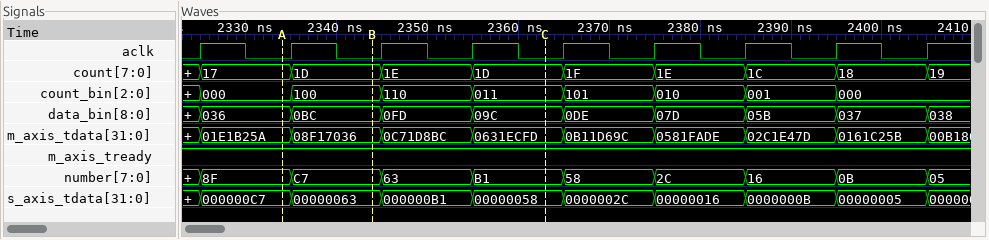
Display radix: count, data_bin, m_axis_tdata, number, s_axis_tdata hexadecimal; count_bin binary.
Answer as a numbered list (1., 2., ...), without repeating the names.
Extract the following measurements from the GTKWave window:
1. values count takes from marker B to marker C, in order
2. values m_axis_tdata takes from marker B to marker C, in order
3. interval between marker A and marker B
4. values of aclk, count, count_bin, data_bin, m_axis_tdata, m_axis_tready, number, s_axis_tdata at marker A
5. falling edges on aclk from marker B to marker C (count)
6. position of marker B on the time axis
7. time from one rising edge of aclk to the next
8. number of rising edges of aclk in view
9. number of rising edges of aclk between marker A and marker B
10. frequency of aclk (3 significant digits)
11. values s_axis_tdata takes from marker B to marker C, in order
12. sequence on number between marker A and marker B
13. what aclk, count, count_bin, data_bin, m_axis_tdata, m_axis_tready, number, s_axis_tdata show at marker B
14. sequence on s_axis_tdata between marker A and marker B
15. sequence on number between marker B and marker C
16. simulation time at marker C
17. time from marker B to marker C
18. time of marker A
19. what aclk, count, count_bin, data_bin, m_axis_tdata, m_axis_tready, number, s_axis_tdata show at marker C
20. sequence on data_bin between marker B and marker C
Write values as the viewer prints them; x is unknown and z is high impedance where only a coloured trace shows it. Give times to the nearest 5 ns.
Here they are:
1. 1D, 1E, 1D
2. 08F17036, 0C71D8BC, 0631ECFD
3. 10 ns
4. aclk=0, count=17, count_bin=000, data_bin=036, m_axis_tdata=01E1B25A, m_axis_tready=1, number=8F, s_axis_tdata=000000C7
5. 2
6. 2345 ns
7. 10 ns
8. 9
9. 1
10. 100 MHz
11. 00000063, 000000B1, 00000058
12. 8F, C7
13. aclk=0, count=1D, count_bin=100, data_bin=0BC, m_axis_tdata=08F17036, m_axis_tready=1, number=C7, s_axis_tdata=00000063
14. 000000C7, 00000063
15. C7, 63, B1
16. 2365 ns
17. 20 ns
18. 2335 ns
19. aclk=0, count=1D, count_bin=011, data_bin=09C, m_axis_tdata=0631ECFD, m_axis_tready=1, number=B1, s_axis_tdata=00000058
20. 0BC, 0FD, 09C
